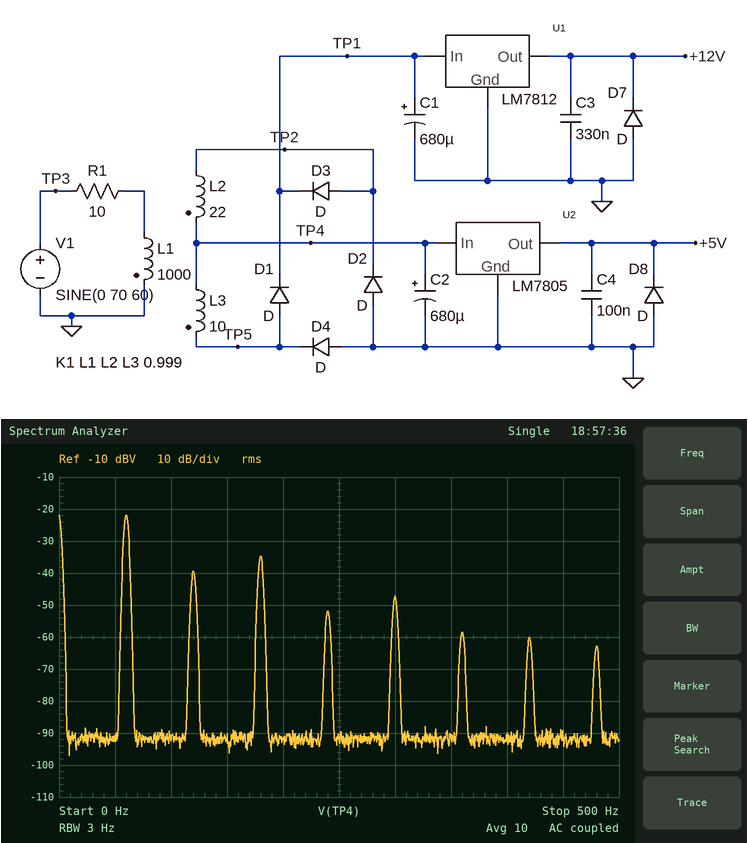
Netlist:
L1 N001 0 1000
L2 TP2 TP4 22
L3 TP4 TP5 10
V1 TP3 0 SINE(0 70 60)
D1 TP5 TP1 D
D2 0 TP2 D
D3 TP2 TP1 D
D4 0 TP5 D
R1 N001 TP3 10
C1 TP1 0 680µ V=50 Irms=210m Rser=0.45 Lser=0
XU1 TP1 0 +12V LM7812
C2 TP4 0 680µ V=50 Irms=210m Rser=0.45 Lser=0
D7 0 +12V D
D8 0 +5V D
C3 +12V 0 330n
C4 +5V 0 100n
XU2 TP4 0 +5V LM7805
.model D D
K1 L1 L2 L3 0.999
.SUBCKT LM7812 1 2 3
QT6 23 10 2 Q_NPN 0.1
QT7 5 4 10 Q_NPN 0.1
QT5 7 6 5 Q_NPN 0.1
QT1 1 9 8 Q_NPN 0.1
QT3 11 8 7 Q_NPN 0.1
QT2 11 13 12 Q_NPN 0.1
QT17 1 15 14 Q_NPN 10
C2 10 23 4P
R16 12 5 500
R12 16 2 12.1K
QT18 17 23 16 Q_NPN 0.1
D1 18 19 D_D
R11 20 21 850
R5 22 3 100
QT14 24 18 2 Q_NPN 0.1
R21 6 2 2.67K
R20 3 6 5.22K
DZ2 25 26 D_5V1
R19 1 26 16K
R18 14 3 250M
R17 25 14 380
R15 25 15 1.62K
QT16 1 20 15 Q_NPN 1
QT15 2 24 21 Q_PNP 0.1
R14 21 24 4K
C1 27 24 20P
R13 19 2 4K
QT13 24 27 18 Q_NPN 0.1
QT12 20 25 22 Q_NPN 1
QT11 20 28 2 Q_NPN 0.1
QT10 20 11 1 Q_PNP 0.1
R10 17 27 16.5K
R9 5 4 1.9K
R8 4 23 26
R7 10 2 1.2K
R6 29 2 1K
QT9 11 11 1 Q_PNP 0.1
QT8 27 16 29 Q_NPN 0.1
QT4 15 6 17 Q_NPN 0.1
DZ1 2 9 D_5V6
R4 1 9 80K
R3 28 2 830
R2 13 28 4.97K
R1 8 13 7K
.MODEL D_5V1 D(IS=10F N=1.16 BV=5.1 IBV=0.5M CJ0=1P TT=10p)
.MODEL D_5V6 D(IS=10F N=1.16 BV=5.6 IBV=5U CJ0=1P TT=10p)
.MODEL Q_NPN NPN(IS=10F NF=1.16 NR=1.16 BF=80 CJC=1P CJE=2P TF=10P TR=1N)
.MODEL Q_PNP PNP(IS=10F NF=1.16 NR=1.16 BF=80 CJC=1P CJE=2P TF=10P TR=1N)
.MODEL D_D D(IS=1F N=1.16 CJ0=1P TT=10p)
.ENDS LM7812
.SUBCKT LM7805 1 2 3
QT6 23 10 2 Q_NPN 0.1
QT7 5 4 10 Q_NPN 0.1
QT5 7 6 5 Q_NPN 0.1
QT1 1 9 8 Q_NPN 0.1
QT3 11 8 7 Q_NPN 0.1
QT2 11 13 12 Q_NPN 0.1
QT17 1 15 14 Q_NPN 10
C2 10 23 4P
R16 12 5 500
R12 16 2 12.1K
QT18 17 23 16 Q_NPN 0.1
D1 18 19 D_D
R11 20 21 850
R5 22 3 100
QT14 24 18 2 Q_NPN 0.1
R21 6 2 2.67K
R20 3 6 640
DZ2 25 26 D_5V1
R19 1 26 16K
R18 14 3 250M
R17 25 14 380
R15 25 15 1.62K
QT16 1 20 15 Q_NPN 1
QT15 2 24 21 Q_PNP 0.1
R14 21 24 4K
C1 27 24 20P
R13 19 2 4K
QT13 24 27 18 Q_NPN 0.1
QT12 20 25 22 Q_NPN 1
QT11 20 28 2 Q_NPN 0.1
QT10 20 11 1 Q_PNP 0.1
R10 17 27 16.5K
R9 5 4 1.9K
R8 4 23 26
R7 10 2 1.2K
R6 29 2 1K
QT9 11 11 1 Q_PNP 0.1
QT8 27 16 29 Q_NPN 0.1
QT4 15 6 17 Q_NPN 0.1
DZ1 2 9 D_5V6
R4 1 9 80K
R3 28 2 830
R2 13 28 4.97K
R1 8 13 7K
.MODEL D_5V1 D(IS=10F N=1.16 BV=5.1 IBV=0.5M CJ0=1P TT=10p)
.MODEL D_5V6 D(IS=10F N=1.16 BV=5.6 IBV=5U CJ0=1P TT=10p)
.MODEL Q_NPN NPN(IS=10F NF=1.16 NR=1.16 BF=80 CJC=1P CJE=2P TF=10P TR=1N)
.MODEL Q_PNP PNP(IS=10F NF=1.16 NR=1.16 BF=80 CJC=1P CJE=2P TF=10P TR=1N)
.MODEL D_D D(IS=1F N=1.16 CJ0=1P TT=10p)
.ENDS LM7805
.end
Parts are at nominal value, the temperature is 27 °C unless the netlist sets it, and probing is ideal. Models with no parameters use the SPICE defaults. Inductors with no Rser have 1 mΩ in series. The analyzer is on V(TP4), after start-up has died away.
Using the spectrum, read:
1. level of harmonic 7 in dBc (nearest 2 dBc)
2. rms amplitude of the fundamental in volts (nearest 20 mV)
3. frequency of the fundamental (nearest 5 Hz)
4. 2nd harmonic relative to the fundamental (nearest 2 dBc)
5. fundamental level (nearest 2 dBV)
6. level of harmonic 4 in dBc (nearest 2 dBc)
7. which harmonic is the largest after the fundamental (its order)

-38 dBc
80 mV
60 Hz
-18 dBc
-22 dBV
-30 dBc
3
